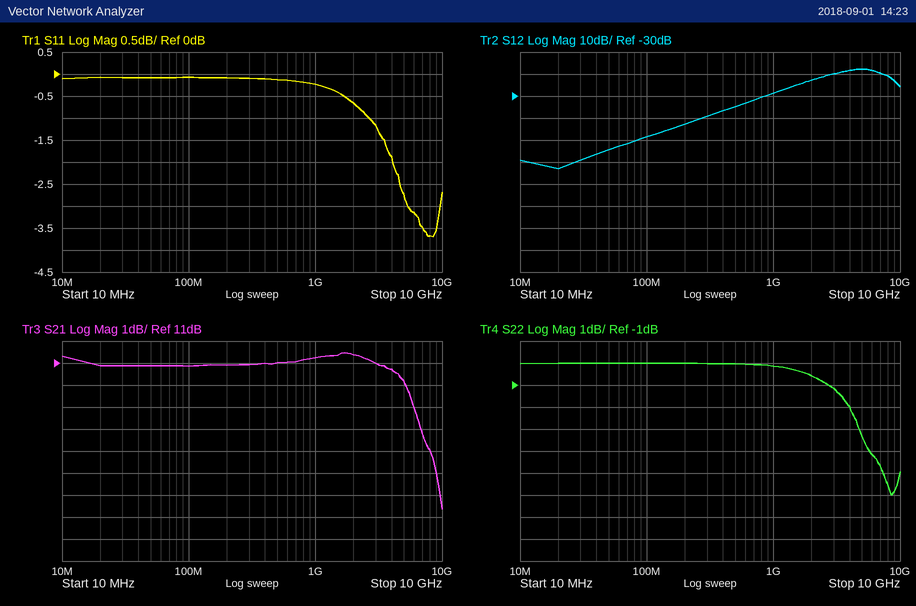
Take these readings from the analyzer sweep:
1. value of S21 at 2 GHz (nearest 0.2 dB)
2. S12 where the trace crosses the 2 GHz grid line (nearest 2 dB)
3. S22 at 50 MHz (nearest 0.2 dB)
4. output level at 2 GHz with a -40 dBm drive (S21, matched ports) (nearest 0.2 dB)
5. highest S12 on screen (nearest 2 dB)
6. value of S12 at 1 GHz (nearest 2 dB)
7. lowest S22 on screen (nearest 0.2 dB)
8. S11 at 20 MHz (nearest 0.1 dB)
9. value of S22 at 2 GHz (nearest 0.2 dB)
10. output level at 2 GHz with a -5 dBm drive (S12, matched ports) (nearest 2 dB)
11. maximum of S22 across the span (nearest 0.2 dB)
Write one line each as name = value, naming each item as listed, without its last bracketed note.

value of S21 at 2 GHz = 11.4 dB
S12 where the trace crosses the 2 GHz grid line = -22 dB
S22 at 50 MHz = 0.0 dB
output level at 2 GHz with a -40 dBm drive (S21, matched ports) = -28.6 dBm
highest S12 on screen = -18 dB
value of S12 at 1 GHz = -28 dB
lowest S22 on screen = -6.0 dB
S11 at 20 MHz = -0.1 dB
value of S22 at 2 GHz = -0.6 dB
output level at 2 GHz with a -5 dBm drive (S12, matched ports) = -28 dBm
maximum of S22 across the span = 0.0 dB
